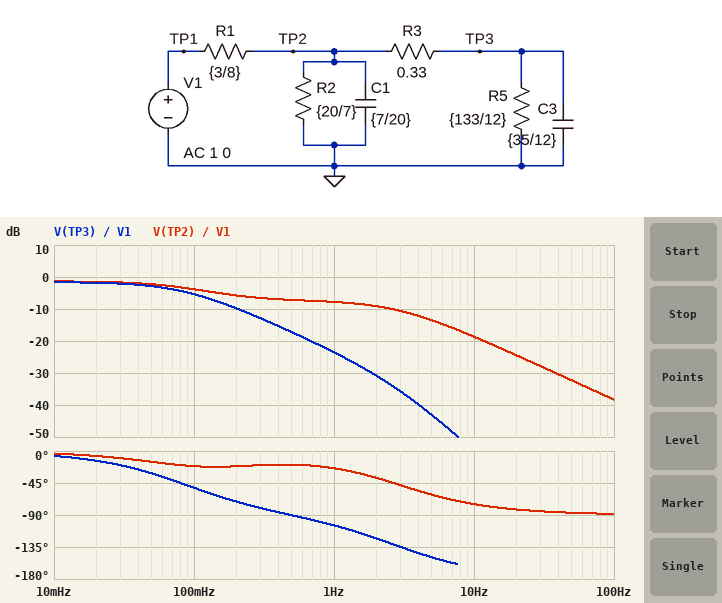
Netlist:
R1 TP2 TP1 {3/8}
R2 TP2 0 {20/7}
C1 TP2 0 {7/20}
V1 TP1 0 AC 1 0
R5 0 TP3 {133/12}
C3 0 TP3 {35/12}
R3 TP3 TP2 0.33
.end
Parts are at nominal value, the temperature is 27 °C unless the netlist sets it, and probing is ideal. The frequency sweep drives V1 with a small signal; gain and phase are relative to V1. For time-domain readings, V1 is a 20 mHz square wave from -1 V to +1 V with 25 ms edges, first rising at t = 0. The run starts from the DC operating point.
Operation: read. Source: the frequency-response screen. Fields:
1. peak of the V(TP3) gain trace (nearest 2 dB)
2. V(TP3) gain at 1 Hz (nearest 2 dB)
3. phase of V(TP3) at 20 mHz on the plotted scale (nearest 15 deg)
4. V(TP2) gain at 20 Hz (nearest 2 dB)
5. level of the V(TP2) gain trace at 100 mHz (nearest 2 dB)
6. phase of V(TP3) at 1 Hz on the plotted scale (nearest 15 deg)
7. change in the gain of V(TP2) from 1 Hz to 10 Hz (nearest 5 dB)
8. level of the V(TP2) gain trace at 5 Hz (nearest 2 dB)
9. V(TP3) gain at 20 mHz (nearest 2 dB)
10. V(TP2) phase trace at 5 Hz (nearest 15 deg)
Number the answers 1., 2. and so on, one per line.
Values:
1. -2 dB
2. -24 dB
3. -15 deg
4. -24 dB
5. -4 dB
6. -105 deg
7. -10 dB
8. -14 dB
9. -2 dB
10. -60 deg
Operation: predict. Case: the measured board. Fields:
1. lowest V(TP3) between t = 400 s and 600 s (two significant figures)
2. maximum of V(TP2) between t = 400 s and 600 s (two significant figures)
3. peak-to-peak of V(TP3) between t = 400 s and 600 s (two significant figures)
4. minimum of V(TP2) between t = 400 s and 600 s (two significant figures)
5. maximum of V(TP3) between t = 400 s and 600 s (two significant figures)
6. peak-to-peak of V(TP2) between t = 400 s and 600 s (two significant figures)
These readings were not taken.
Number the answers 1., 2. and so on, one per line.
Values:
1. -830 mV
2. 860 mV
3. 1.7 V
4. -860 mV
5. 830 mV
6. 1.7 V
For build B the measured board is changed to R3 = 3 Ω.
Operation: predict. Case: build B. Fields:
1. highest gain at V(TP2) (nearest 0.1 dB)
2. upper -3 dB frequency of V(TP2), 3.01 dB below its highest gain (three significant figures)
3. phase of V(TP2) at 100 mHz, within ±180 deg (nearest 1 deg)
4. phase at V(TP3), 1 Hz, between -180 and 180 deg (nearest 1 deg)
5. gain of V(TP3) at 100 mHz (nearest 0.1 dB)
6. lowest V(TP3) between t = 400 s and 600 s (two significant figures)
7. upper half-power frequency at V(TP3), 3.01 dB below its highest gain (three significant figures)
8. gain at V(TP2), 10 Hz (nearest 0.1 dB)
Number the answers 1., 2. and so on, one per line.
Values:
1. -1.3 dB
2. 1.27 Hz
3. -5 deg
4. -122 deg
5. -17.0 dB
6. -630 mV
7. 21.3 mHz
8. -18.4 dB
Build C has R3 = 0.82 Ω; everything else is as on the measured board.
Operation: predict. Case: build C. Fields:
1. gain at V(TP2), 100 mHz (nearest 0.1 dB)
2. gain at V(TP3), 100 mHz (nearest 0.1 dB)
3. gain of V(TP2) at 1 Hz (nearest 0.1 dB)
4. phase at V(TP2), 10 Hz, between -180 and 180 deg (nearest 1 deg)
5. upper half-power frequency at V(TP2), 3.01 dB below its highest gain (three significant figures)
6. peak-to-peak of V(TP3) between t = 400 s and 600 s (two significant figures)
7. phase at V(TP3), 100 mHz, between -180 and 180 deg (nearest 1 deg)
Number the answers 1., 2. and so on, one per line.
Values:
1. -3.4 dB
2. -8.7 dB
3. -5.1 dB
4. -79 deg
5. 480 mHz
6. 1.6 V
7. -66 deg
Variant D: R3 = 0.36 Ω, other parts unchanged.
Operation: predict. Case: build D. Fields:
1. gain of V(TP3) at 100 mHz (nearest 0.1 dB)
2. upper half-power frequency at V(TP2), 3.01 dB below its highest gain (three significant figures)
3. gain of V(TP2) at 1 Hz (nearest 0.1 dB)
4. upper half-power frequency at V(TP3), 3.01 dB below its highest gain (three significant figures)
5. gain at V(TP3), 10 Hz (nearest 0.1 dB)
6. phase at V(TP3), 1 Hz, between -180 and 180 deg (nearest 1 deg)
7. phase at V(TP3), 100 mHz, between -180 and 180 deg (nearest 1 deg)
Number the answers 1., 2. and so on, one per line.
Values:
1. -5.6 dB
2. 120 mHz
3. -7.5 dB
4. 81.4 mHz
5. -55.0 dB
6. -106 deg
7. -53 deg
